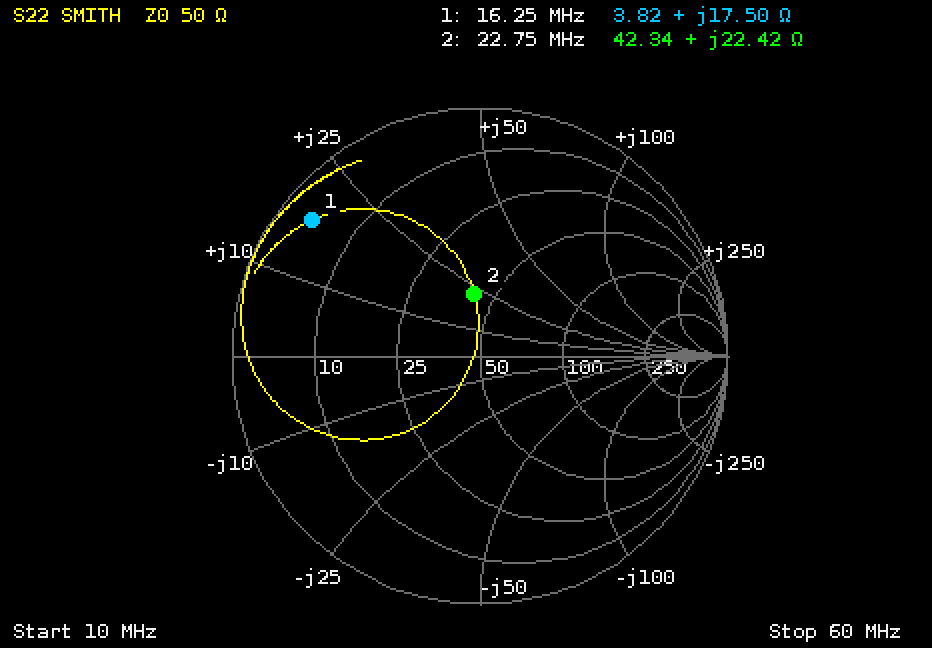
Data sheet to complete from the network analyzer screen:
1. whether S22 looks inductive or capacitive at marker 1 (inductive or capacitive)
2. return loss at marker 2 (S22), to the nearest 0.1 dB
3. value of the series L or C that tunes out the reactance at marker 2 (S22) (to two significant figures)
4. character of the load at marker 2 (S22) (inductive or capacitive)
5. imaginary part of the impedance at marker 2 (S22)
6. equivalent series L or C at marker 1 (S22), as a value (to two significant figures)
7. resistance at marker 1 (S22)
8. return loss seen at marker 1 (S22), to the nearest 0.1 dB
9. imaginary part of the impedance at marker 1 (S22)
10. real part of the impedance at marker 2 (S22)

inductive
12.1 dB
310 pF
inductive
+22.42 Ω
170 nH
3.82 Ω
1.2 dB
+17.50 Ω
42.34 Ω
